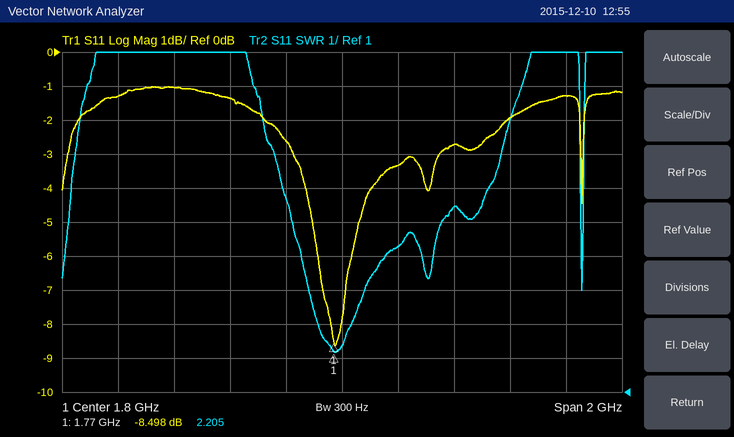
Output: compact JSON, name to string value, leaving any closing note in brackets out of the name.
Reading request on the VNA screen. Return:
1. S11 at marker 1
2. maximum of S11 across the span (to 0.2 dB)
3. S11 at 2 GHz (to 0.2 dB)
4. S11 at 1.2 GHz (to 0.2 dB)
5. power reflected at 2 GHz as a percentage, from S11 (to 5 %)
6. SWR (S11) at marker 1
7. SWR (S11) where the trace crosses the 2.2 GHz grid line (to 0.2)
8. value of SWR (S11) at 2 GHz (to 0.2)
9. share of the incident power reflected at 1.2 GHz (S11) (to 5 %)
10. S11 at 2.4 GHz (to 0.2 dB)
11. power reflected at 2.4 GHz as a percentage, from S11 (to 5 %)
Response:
{"S11 at marker 1": "-8.498 dB", "maximum of S11 across the span": "-1.0 dB", "S11 at 2 GHz": "-3.4 dB", "S11 at 1.2 GHz": "-1.0 dB", "power reflected at 2 GHz as a percentage, from S11": "45 %", "SWR (S11) at marker 1": "2.205", "SWR (S11) where the trace crosses the 2.2 GHz grid line": "6.4", "value of SWR (S11) at 2 GHz": "5.2", "share of the incident power reflected at 1.2 GHz (S11)": "80 %", "S11 at 2.4 GHz": "-2.0 dB", "power reflected at 2.4 GHz as a percentage, from S11": "65 %"}
